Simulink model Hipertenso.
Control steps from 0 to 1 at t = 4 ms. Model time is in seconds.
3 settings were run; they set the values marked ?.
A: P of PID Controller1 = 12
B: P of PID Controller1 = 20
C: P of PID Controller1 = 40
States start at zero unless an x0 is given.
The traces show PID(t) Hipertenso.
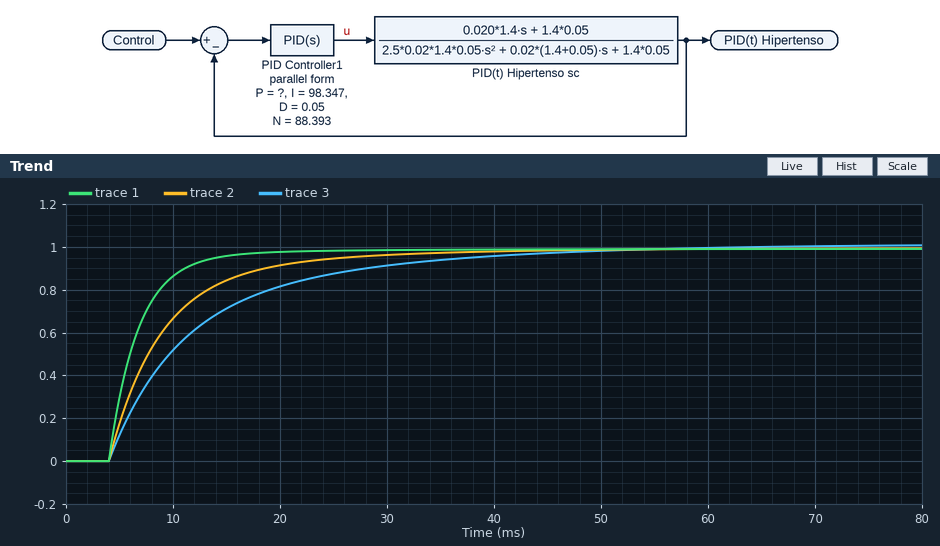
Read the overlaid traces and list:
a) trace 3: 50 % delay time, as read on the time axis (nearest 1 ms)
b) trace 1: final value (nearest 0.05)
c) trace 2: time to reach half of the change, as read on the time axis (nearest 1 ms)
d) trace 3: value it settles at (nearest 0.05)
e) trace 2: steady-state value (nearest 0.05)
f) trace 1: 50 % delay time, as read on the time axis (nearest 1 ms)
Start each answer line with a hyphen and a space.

- 10 ms
- 1.00
- 8 ms
- 1.00
- 1.00
- 6 ms
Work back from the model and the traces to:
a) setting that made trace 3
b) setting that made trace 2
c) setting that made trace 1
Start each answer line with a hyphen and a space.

- A
- B
- C
